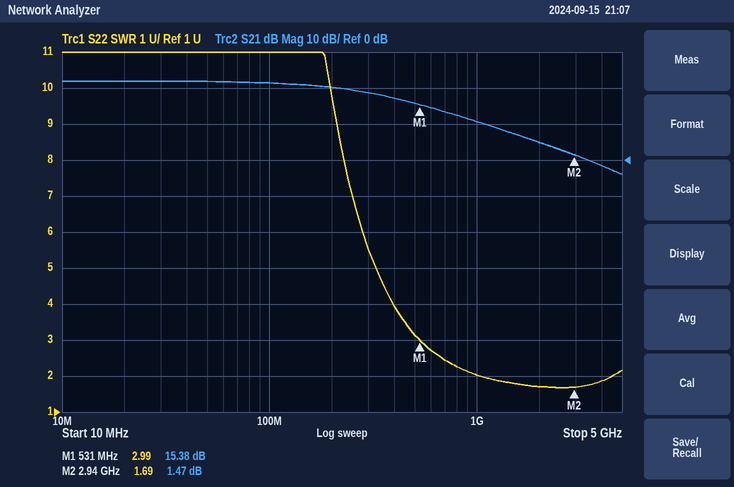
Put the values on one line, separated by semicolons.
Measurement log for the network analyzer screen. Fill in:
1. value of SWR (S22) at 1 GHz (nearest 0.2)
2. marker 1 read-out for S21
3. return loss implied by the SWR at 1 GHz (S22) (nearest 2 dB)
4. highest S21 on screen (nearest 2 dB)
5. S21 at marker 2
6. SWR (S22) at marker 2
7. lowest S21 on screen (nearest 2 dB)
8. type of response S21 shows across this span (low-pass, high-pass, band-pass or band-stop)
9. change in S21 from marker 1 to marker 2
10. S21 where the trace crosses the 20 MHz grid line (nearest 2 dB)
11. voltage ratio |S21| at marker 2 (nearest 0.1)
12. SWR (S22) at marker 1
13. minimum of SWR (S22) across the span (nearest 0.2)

2.0; 15.38 dB; 10 dB; 22 dB; 1.47 dB; 1.69; -4 dB; low-pass; -13.91 dB; 22 dB; 1.2; 2.99; 1.6
